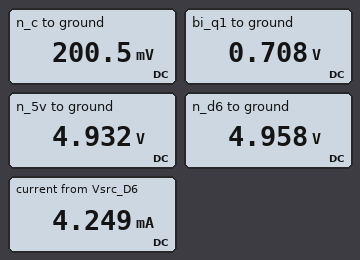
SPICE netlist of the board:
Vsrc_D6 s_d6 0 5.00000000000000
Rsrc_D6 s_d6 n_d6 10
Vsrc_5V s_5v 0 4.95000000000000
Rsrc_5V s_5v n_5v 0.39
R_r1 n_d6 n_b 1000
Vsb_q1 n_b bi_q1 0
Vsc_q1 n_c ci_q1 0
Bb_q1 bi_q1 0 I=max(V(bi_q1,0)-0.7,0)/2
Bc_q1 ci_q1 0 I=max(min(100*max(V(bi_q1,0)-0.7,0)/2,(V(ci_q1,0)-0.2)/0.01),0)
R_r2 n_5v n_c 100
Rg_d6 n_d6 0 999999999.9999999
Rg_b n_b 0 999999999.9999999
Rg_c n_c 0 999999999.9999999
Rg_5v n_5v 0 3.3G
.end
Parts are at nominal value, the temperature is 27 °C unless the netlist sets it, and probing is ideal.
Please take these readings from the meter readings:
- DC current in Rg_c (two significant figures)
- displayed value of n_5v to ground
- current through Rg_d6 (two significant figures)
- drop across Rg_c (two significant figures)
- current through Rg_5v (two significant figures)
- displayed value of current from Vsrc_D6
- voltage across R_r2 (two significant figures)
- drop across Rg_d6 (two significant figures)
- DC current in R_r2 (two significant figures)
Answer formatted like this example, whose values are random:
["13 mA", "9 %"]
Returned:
["200 pA", "4.932 V", "5.0 nA", "200 mV", "1.5 nA", "4.249 mA", "4.7 V", "5.0 V", "47 mA"]
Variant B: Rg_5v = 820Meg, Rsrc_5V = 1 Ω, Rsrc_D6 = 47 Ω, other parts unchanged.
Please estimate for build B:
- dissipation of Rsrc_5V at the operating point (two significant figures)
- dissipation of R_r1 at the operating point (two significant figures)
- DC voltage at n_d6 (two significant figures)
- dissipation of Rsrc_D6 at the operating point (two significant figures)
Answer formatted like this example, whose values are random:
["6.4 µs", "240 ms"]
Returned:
["2.2 mW", "17 mW", "4.8 V", "790 µW"]
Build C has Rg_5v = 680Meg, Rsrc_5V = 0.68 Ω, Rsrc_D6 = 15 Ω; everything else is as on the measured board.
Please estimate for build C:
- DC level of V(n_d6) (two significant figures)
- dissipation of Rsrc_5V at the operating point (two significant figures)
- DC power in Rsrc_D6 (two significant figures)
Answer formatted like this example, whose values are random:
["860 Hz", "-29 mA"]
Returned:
["4.9 V", "1.5 mW", "270 µW"]
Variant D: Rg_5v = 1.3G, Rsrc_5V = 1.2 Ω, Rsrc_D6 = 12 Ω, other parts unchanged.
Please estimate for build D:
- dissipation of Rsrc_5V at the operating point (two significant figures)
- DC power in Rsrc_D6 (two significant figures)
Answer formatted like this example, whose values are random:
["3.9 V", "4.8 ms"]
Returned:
["2.6 mW", "220 µW"]
